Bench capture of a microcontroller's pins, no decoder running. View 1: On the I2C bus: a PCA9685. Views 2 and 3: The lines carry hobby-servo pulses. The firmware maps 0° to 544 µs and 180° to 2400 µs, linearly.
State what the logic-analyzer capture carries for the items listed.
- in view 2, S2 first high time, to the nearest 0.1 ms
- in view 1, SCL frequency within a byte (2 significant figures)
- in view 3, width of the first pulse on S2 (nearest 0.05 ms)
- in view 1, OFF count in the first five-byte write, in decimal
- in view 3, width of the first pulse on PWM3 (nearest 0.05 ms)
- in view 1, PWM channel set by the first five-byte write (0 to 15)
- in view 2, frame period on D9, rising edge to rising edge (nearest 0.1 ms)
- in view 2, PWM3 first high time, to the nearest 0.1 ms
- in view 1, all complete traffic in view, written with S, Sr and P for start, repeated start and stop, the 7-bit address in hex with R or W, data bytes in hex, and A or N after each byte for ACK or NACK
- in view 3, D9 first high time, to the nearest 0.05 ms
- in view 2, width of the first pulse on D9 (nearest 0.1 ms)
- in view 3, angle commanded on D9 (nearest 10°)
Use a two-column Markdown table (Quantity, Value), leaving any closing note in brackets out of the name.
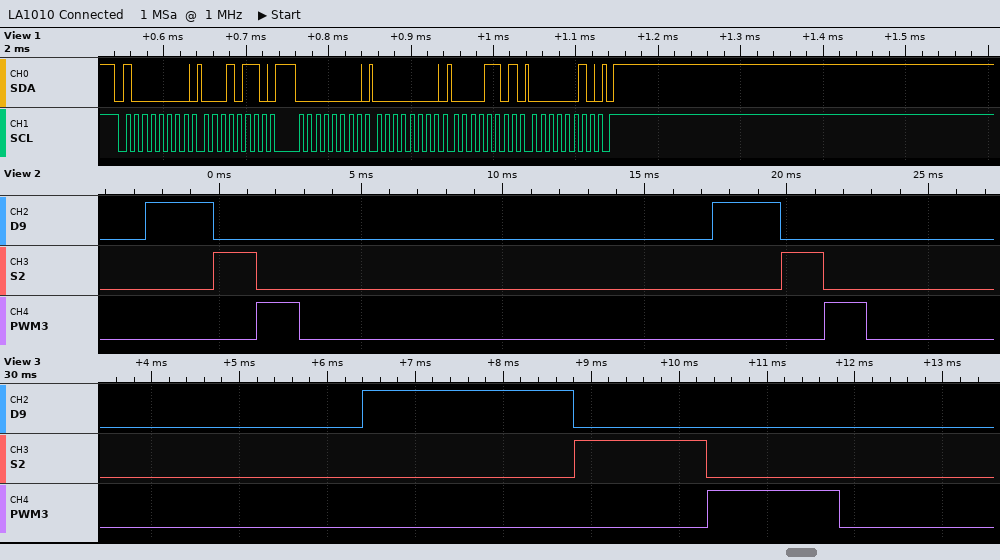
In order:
| Quantity | Value |
|---|---|
| in view 2, S2 first high time, to the nearest 0.1 ms | 1.5 ms |
| in view 1, SCL frequency within a byte | 100 kHz |
| in view 3, width of the first pulse on S2 | 1.50 ms |
| in view 1, OFF count in the first five-byte write, in decimal | 525 |
| in view 3, width of the first pulse on PWM3 | 1.50 ms |
| in view 1, PWM channel set by the first five-byte write | 4 |
| in view 2, frame period on D9, rising edge to rising edge | 20.0 ms |
| in view 2, PWM3 first high time, to the nearest 0.1 ms | 1.5 ms |
| in view 1, all complete traffic in view, written with S, Sr and P for start, repeated start and stop, the 7-bit address in hex with R or W, data bytes in hex, and A or N after each byte for ACK or NACK | S 40W A 16 A 00 A 00 A 0D A 02 A P |
| in view 3, D9 first high time, to the nearest 0.05 ms | 2.40 ms |
| in view 2, width of the first pulse on D9 | 2.4 ms |
| in view 3, angle commanded on D9 | 180° |
